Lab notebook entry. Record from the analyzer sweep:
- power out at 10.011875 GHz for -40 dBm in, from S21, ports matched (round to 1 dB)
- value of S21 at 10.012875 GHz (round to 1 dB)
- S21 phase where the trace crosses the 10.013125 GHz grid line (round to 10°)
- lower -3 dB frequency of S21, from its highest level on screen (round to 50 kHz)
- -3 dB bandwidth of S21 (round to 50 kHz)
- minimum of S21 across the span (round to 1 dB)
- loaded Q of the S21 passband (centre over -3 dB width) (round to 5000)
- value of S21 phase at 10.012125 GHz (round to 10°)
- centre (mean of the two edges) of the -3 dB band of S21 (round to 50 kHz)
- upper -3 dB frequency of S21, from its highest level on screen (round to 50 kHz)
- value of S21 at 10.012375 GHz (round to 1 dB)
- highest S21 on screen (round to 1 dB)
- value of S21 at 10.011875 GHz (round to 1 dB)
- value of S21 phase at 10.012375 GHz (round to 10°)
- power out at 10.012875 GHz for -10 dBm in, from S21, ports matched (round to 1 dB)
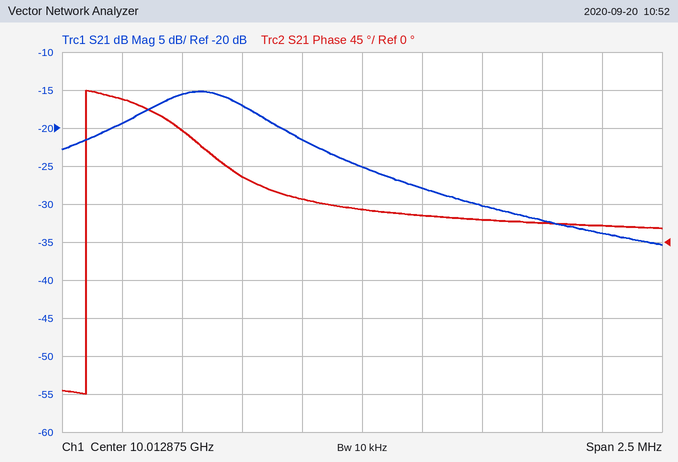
-59 dBm
-25 dB
30°
10.01195 GHz
500 kHz
-35 dB
20000
130°
10.01220 GHz
10.01245 GHz
-17 dB
-15 dB
-19 dB
80°
-35 dBm
